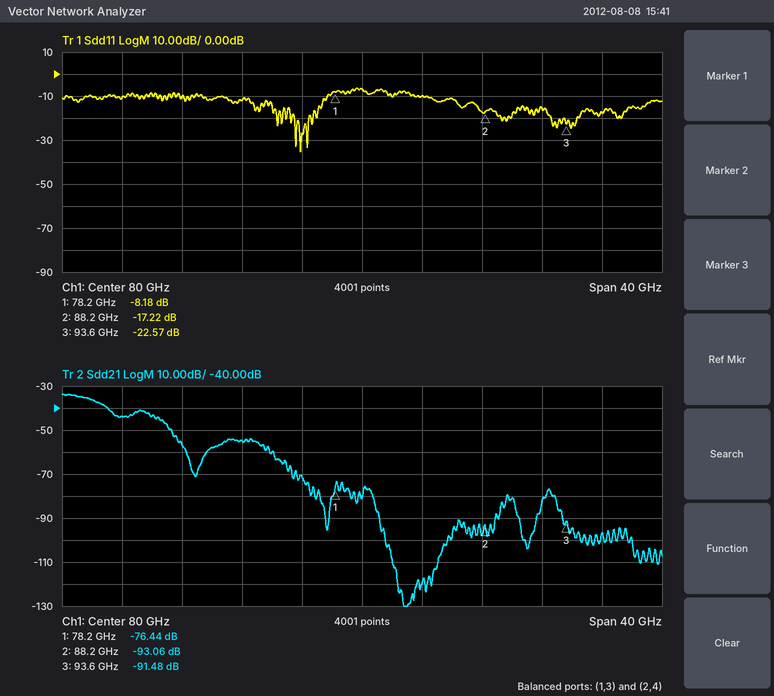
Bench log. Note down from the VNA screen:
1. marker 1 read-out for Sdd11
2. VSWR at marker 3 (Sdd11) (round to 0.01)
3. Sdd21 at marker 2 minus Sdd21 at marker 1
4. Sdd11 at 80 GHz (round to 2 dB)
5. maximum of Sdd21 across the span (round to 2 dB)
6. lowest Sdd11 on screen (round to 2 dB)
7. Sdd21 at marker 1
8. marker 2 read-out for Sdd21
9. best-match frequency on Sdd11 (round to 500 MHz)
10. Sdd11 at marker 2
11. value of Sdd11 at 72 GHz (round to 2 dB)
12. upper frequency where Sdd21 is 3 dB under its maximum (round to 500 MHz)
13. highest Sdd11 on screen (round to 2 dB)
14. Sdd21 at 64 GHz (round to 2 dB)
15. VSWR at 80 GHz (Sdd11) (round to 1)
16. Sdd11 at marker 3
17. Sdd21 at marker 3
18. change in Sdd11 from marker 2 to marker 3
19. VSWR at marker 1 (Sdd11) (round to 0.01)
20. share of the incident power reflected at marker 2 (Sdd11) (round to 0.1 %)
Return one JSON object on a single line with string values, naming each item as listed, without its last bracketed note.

{"marker 1 read-out for Sdd11": "-8.18 dB", "VSWR at marker 3 (Sdd11)": "1.16", "Sdd21 at marker 2 minus Sdd21 at marker 1": "-16.62 dB", "Sdd11 at 80 GHz": "-6 dB", "maximum of Sdd21 across the span": "-34 dB", "lowest Sdd11 on screen": "-36 dB", "Sdd21 at marker 1": "-76.44 dB", "marker 2 read-out for Sdd21": "-93.06 dB", "best-match frequency on Sdd11": "76.0 GHz", "Sdd11 at marker 2": "-17.22 dB", "value of Sdd11 at 72 GHz": "-12 dB", "upper frequency where Sdd21 is 3 dB under its maximum": "62.0 GHz", "highest Sdd11 on screen": "-6 dB", "Sdd21 at 64 GHz": "-44 dB", "VSWR at 80 GHz (Sdd11)": "3", "Sdd11 at marker 3": "-22.57 dB", "Sdd21 at marker 3": "-91.48 dB", "change in Sdd11 from marker 2 to marker 3": "-5.35 dB", "VSWR at marker 1 (Sdd11)": "2.28", "share of the incident power reflected at marker 2 (Sdd11)": "1.9 %"}
